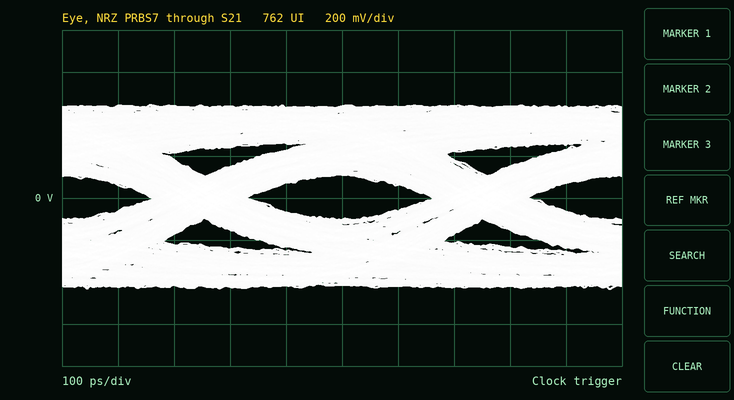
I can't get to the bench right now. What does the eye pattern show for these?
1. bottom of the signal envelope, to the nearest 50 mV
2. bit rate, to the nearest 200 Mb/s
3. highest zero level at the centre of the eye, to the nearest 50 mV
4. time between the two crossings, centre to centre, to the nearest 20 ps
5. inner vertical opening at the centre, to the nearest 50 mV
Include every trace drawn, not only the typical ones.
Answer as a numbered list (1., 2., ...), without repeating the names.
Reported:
1. -450 mV
2. 2.0 Gb/s
3. -100 mV
4. 500 ps
5. 200 mV
